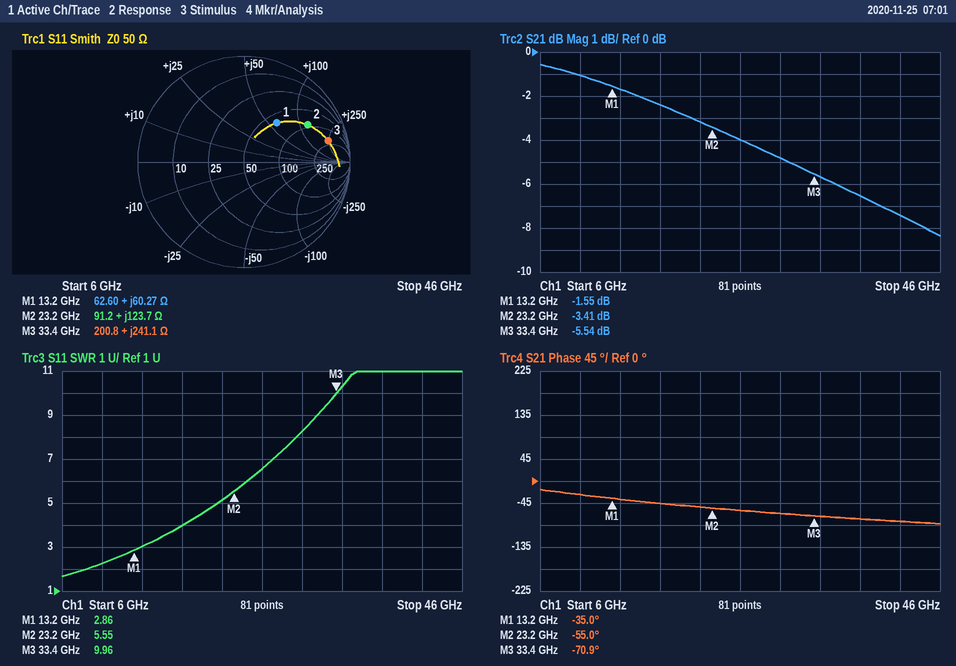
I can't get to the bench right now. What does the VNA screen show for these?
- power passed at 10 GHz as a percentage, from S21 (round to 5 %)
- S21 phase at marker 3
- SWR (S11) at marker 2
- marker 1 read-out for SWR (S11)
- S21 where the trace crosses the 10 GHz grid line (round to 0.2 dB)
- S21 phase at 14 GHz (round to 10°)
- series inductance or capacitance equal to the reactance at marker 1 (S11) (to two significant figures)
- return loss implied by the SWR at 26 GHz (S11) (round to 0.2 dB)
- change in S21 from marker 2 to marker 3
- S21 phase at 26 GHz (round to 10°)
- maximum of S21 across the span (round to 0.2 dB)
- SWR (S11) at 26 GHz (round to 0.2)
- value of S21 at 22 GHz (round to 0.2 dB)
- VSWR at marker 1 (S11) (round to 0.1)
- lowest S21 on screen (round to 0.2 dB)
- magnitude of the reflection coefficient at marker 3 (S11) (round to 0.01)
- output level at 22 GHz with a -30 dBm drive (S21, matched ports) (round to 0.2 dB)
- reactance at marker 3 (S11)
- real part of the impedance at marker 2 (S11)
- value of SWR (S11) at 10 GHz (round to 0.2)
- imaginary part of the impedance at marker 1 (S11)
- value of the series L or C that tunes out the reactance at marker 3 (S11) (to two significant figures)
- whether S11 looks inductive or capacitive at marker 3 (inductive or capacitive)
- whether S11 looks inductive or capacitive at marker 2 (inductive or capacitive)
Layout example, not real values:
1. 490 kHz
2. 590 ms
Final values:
1. 80 %
2. -70.9°
3. 5.55
4. 2.86
5. -1.0 dB
6. -40°
7. 730 pH
8. 2.6 dB
9. -2.13 dB
10. -60°
11. -0.6 dB
12. 6.6
13. -3.2 dB
14. 2.9
15. -8.4 dB
16. 0.82
17. -33.2 dBm
18. +241.1 Ω
19. 91.2 Ω
20. 2.2
21. +60.27 Ω
22. 20 fF
23. inductive
24. inductive
